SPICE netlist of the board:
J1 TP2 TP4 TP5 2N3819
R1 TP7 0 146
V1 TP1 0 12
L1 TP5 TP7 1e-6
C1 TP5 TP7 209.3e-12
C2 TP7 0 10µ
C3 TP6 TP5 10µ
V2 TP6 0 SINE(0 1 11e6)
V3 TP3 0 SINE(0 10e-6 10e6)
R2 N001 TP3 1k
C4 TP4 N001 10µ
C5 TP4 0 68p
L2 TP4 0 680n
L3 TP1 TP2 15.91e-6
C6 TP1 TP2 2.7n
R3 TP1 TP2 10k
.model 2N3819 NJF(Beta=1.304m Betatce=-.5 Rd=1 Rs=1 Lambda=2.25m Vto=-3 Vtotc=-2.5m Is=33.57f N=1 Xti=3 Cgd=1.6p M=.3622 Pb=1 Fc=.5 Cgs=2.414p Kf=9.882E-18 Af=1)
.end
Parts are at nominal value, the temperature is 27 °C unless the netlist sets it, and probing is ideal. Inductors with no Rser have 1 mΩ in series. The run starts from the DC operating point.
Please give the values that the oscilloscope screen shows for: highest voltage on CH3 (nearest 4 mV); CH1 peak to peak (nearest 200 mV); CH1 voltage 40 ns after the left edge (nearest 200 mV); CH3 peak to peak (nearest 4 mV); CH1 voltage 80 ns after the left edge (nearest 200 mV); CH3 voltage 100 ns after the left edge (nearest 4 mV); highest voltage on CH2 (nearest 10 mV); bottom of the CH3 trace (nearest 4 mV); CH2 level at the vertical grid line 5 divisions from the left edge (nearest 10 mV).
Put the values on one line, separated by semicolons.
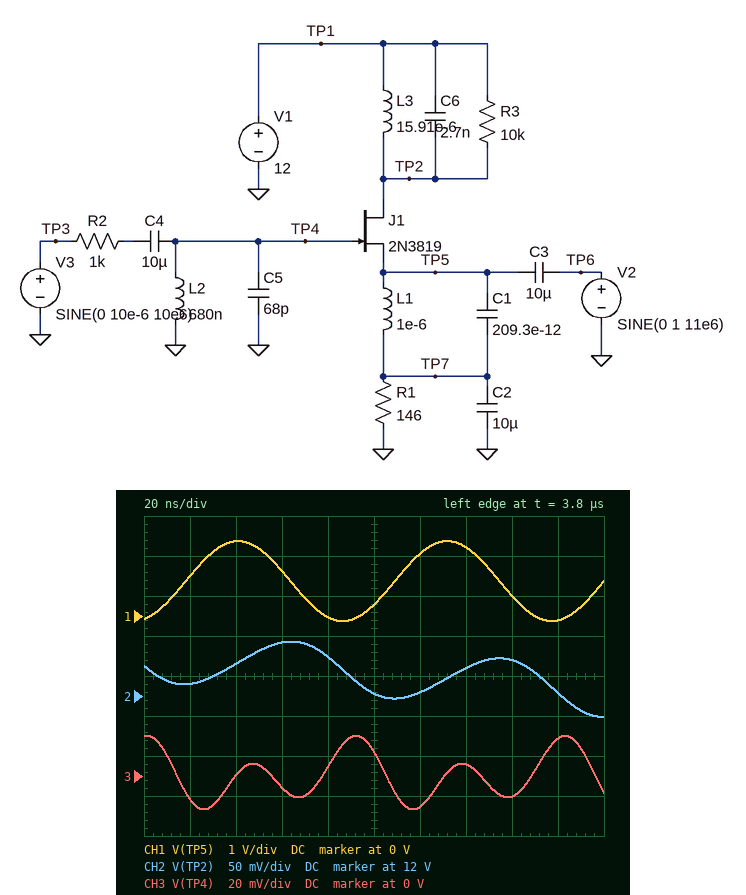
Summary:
20 mV; 2.0 V; 1.8 V; 36 mV; 0 V; 12 mV; 12.07 V; -16 mV; 12.00 V
